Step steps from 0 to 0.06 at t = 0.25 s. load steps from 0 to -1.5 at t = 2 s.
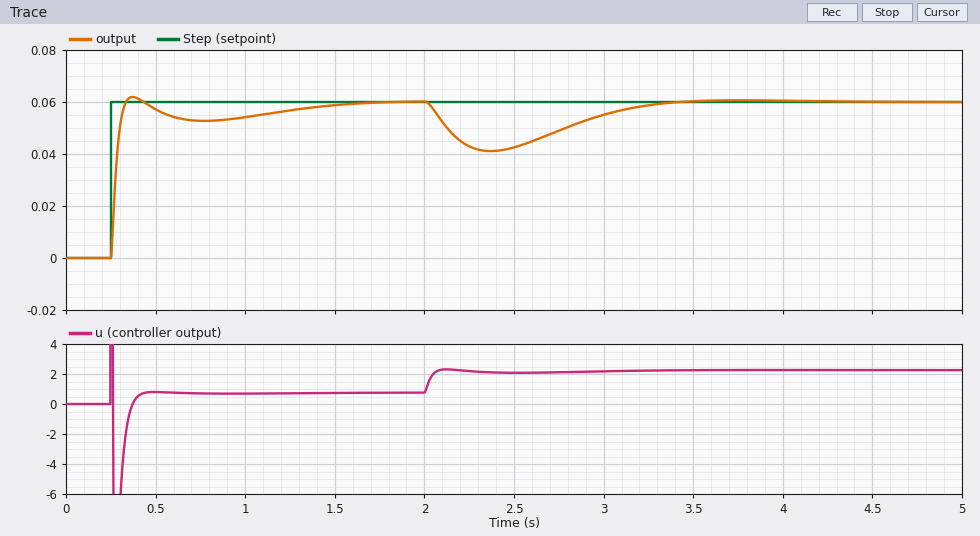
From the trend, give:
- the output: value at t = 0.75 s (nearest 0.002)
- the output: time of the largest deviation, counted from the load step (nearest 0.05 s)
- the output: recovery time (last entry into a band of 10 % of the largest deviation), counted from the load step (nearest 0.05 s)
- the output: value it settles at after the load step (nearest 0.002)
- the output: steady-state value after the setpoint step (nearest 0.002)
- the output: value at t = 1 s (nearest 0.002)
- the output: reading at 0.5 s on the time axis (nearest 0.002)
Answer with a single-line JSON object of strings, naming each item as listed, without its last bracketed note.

{"the output: value at t = 0.75 s": "0.052", "the output: time of the largest deviation, counted from the load step": "0.35 s", "the output: recovery time (last entry into a band of 10 % of the largest deviation), counted from the load step": "1.20 s", "the output: value it settles at after the load step": "0.060", "the output: steady-state value after the setpoint step": "0.060", "the output: value at t = 1 s": "0.054", "the output: reading at 0.5 s on the time axis": "0.058"}
